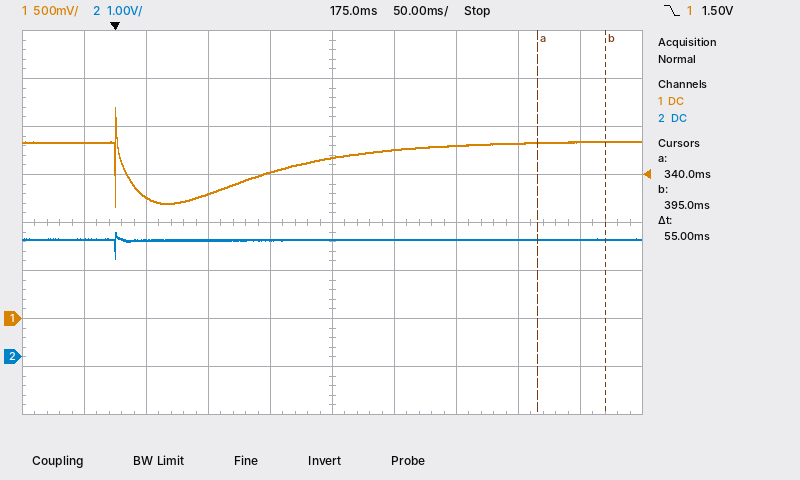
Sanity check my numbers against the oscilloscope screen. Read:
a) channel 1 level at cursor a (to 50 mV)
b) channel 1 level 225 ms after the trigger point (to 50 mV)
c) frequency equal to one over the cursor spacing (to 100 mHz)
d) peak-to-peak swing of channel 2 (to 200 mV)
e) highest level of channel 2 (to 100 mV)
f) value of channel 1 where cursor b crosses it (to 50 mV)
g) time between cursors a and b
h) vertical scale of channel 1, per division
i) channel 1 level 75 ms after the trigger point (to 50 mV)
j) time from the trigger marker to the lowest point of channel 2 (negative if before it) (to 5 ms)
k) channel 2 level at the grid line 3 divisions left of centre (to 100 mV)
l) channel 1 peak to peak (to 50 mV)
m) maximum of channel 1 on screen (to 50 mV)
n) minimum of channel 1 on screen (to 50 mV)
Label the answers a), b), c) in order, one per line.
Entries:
a) 1.85 V
b) 1.75 V
c) 18.2 Hz
d) 600 mV
e) 2.6 V
f) 1.85 V
g) 55 ms
h) 500 mV
i) 1.30 V
j) 0 ms
k) 2.4 V
l) 1.05 V
m) 2.20 V
n) 1.15 V
